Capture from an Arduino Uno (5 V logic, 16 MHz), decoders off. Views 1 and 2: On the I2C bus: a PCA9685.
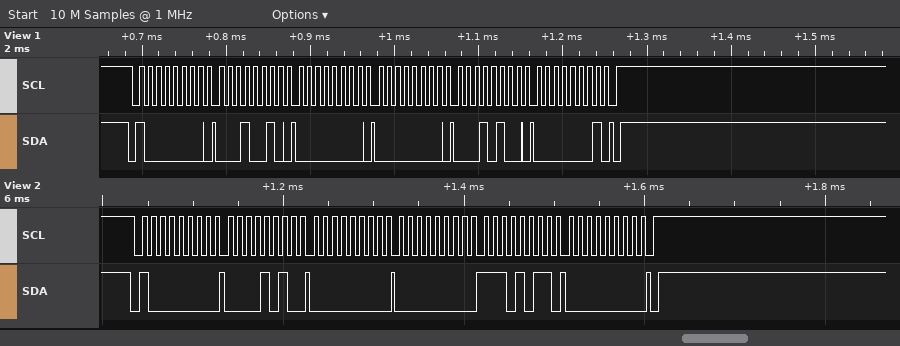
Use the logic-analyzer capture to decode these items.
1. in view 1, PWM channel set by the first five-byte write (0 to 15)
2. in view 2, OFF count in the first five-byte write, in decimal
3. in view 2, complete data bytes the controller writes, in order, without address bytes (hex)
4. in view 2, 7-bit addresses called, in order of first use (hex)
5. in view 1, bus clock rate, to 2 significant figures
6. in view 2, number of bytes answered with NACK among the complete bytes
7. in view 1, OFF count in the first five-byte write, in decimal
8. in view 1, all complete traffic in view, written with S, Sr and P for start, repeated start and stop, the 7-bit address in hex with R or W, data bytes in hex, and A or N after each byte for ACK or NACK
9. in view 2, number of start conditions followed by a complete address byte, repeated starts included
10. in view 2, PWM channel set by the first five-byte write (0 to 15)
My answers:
3
235
0A 00 00 EB 00
0x40
100 kHz
0
276
S 40W A 12 A 00 A 00 A 14 A 01 A P
1
1
